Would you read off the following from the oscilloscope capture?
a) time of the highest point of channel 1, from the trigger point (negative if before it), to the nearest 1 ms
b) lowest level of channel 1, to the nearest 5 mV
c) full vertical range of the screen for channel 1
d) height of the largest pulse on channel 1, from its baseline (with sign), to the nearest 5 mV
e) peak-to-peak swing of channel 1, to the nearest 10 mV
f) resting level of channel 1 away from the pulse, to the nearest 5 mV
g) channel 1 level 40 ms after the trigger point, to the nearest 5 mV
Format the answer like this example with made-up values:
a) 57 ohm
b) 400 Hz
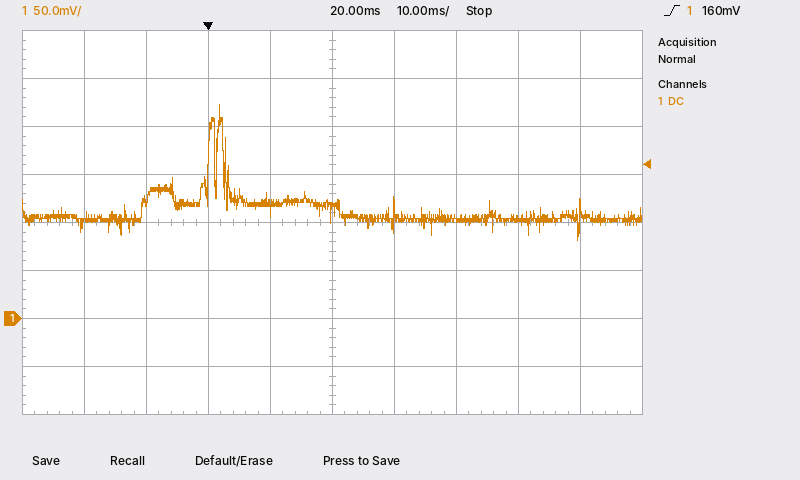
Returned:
a) +2 ms
b) 80 mV
c) 400 mV
d) +120 mV
e) 140 mV
f) 105 mV
g) 105 mV
